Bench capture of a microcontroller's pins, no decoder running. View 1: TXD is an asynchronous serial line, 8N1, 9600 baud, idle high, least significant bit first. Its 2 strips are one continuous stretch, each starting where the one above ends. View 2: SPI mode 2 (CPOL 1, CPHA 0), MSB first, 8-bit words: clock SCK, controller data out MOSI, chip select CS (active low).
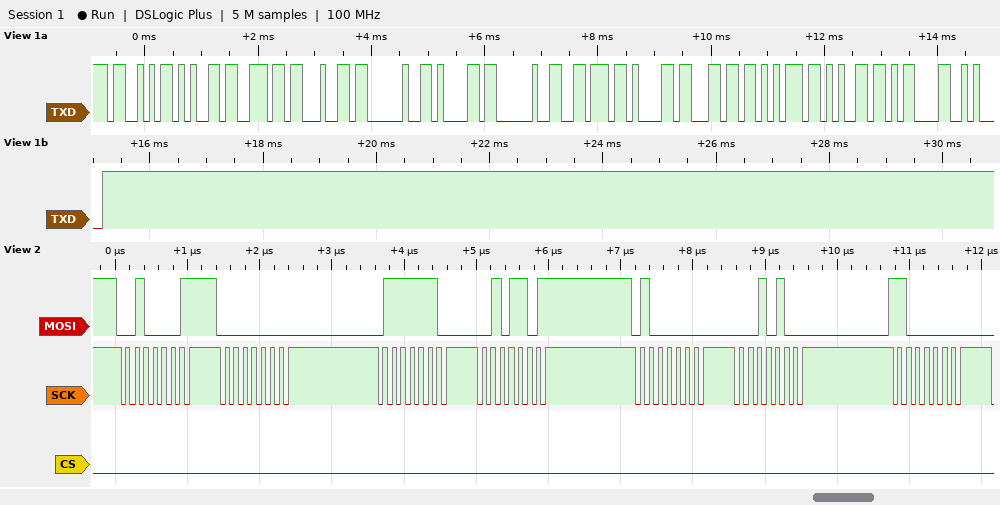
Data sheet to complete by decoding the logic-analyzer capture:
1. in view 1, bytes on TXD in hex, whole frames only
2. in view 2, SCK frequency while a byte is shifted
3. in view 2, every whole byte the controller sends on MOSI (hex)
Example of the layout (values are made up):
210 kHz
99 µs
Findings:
53 65 6E 64 20 61 20 76 61 6C 75 65 0D 0A
8 MHz
21 00 7E 2D 40 14 C0
